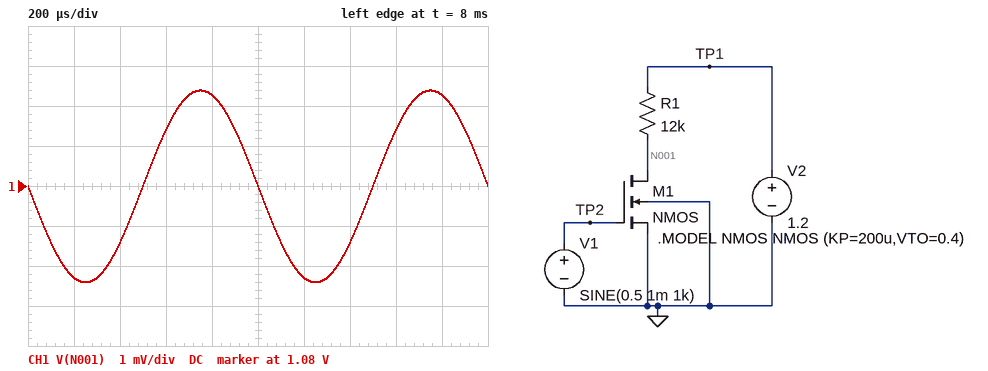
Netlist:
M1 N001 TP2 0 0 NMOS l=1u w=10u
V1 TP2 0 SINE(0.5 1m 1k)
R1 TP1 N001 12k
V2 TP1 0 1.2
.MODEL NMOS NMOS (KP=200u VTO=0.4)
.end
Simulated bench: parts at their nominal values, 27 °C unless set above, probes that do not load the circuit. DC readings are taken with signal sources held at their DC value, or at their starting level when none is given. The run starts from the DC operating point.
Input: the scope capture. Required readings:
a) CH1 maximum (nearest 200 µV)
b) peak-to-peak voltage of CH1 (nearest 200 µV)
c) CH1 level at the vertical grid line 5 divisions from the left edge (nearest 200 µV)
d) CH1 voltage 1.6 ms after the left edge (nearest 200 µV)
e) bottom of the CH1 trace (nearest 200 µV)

1.0824 V
4.8 mV
1.0800 V
1.0814 V
1.0776 V
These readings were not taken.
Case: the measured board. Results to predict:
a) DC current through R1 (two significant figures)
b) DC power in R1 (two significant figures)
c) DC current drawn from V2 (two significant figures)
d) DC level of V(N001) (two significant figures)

10 µA
1.2 µW
10 µA
1.1 V
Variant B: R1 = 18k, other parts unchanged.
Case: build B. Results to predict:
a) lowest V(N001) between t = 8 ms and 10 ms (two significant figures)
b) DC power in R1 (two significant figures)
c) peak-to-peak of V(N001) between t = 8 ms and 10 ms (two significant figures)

1.0 V
1.8 µW
7.2 mV
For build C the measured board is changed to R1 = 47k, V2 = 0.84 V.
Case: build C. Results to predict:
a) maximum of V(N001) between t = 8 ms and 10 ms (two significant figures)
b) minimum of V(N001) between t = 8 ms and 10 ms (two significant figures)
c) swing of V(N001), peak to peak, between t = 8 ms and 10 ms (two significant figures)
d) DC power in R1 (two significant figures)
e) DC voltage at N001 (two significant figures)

380 mV
360 mV
19 mV
4.7 µW
370 mV
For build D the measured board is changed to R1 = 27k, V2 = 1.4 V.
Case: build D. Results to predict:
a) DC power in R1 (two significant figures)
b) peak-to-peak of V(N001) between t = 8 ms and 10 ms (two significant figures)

2.7 µW
11 mV
